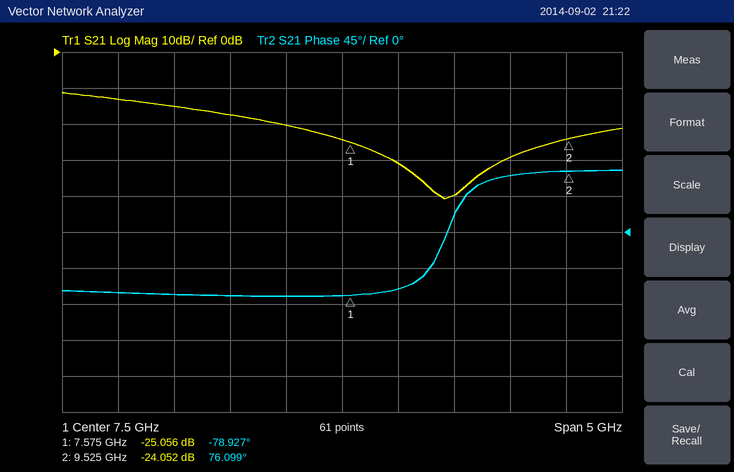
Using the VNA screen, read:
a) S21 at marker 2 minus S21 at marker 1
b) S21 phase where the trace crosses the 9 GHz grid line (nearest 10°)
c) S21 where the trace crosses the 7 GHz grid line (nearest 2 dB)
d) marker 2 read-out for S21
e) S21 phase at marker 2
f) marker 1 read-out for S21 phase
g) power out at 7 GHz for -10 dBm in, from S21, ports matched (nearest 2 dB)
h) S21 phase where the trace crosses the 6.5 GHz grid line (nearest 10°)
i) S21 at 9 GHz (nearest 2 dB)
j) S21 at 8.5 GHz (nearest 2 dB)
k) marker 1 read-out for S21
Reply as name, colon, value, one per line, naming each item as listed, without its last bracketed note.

S21 at marker 2 minus S21 at marker 1: 1.004 dB
S21 phase where the trace crosses the 9 GHz grid line: 70°
S21 where the trace crosses the 7 GHz grid line: -20 dB
marker 2 read-out for S21: -24.052 dB
S21 phase at marker 2: 76.099°
marker 1 read-out for S21 phase: -78.927°
power out at 7 GHz for -10 dBm in, from S21, ports matched: -30 dBm
S21 phase where the trace crosses the 6.5 GHz grid line: -80°
S21 at 9 GHz: -30 dB
S21 at 8.5 GHz: -40 dB
marker 1 read-out for S21: -25.056 dB
